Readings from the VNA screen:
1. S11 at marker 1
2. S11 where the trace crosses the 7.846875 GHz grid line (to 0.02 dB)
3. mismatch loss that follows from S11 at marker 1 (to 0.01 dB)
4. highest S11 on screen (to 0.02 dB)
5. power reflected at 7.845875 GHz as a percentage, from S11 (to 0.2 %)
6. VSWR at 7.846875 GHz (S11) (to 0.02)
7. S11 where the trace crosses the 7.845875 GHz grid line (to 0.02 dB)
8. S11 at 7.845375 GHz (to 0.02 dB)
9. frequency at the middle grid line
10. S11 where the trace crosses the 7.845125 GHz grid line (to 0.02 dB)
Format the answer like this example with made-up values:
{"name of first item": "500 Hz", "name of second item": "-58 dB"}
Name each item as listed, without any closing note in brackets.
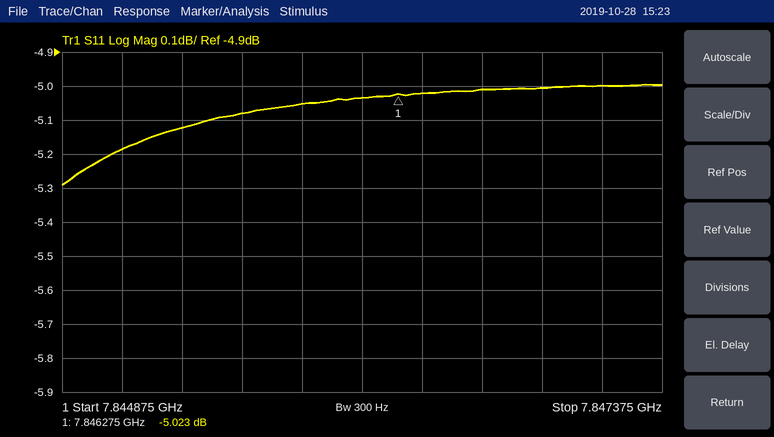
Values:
{"S11 at marker 1": "-5.023 dB", "S11 where the trace crosses the 7.846875 GHz grid line": "-5.00 dB", "mismatch loss that follows from S11 at marker 1": "1.64 dB", "highest S11 on screen": "-5.00 dB", "power reflected at 7.845875 GHz as a percentage, from S11": "31.2 %", "VSWR at 7.846875 GHz (S11)": "3.56", "S11 where the trace crosses the 7.845875 GHz grid line": "-5.06 dB", "S11 at 7.845375 GHz": "-5.12 dB", "frequency at the middle grid line": "7.846125 GHz", "S11 where the trace crosses the 7.845125 GHz grid line": "-5.18 dB"}
